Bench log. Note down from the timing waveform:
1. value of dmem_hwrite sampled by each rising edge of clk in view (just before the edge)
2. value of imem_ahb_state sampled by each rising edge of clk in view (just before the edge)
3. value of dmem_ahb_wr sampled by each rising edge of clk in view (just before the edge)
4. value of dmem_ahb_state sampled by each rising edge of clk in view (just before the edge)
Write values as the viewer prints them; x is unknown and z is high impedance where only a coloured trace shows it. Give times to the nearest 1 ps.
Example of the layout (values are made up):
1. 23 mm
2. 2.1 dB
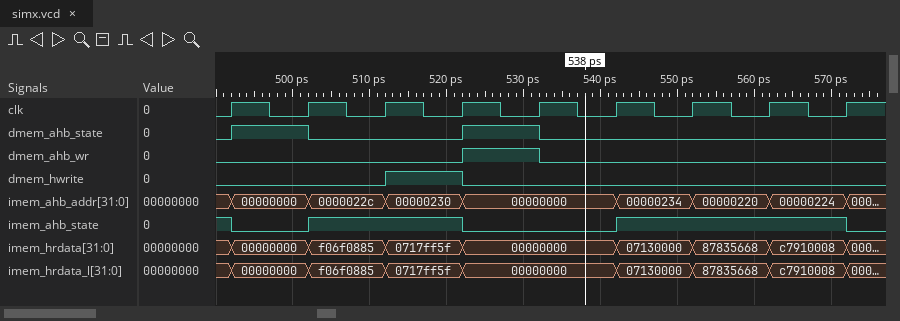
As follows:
1. 0 0 0 1 0 0 0 0 0
2. 1 0 1 1 0 0 1 1 1
3. 0 0 0 0 1 0 0 0 0
4. 0 1 0 0 1 0 0 0 0
